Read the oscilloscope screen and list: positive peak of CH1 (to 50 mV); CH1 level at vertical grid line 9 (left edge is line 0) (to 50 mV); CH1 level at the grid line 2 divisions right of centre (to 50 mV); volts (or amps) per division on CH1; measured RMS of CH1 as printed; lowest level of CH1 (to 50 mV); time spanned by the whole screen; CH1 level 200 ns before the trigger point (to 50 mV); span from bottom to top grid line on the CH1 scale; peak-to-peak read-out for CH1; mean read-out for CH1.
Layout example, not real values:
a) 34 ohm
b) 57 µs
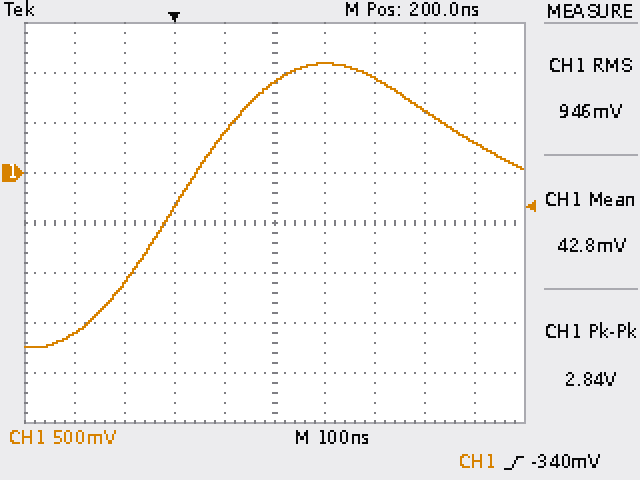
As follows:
a) 1.10 V
b) 300 mV
c) 950 mV
d) 500 mV
e) 946 mV
f) -1.75 V
g) 1 µs
h) -1.60 V
i) 4 V
j) 2.84 V
k) 42.8 mV
